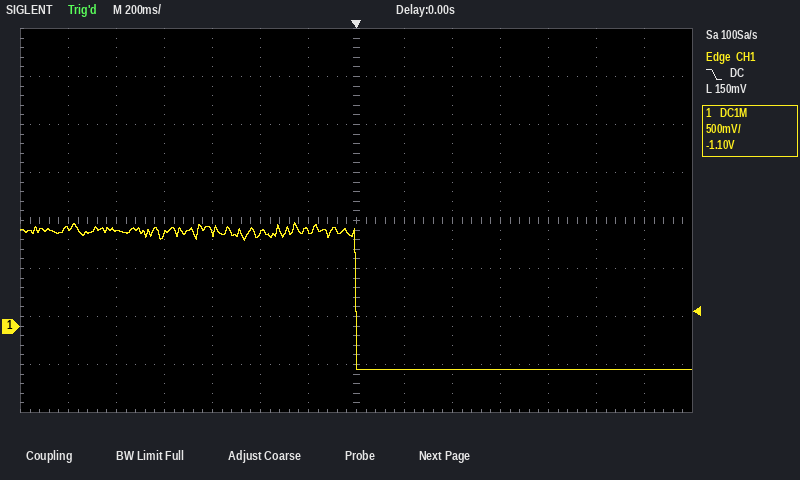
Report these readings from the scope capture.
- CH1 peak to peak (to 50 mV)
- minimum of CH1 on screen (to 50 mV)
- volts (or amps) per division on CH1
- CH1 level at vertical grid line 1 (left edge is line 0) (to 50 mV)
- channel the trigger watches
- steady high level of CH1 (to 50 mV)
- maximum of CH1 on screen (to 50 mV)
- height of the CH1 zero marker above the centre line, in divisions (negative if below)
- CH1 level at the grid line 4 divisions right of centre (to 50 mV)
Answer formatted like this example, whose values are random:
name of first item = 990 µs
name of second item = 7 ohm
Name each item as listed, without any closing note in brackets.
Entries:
CH1 peak to peak = 1.55 V
minimum of CH1 on screen = -450 mV
volts (or amps) per division on CH1 = 500 mV
CH1 level at vertical grid line 1 (left edge is line 0) = 1.00 V
channel the trigger watches = CH1
steady high level of CH1 = 1.00 V
maximum of CH1 on screen = 1.10 V
height of the CH1 zero marker above the centre line, in divisions = -2.2 div
CH1 level at the grid line 4 divisions right of centre = -450 mV
